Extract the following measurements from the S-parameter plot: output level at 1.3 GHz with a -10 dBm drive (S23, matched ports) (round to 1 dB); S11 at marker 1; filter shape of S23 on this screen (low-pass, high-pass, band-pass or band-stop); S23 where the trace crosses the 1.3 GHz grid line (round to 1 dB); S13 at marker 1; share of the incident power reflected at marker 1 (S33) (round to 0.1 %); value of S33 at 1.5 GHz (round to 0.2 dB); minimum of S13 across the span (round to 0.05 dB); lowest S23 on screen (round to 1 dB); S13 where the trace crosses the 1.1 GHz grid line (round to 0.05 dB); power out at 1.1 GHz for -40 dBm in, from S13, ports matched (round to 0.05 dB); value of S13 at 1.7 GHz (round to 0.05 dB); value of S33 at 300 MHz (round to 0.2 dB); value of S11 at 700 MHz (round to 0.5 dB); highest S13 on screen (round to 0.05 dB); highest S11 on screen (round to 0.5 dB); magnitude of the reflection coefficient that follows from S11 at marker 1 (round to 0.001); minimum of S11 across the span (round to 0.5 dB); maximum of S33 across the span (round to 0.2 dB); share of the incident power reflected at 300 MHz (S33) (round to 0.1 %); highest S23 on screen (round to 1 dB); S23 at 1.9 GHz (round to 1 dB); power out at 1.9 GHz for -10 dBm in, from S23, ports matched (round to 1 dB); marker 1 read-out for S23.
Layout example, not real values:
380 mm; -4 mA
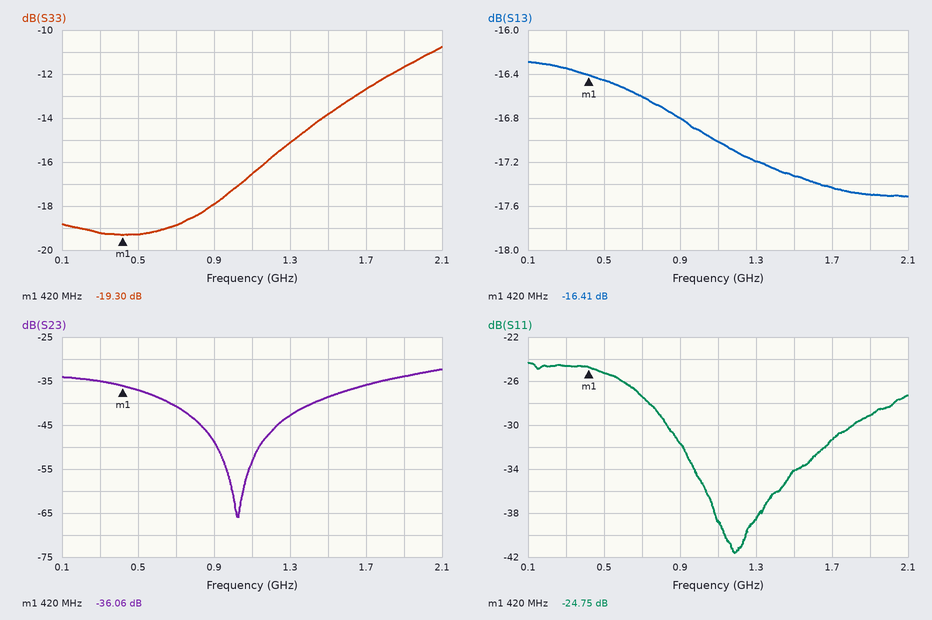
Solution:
-53 dBm; -24.75 dB; band-stop; -43 dB; -16.41 dB; 1.2 %; -13.8 dB; -17.50 dB; -66 dB; -17.00 dB; -57.00 dBm; -17.45 dB; -19.2 dB; -27.5 dB; -16.30 dB; -24.5 dB; 0.058; -41.5 dB; -10.8 dB; 1.2 %; -32 dB; -34 dB; -44 dBm; -36.06 dB
